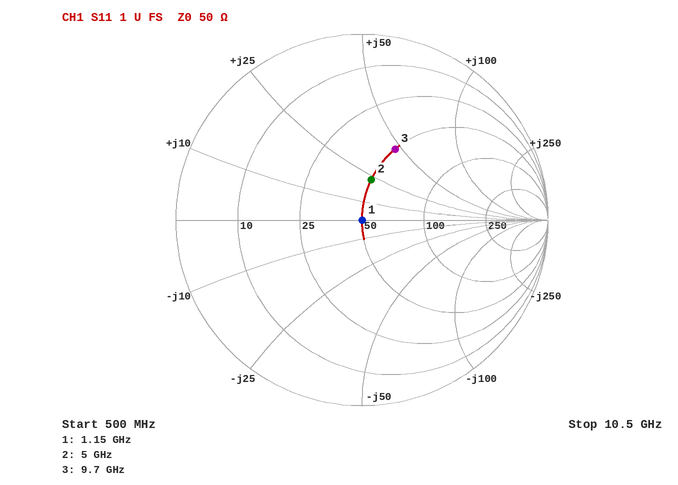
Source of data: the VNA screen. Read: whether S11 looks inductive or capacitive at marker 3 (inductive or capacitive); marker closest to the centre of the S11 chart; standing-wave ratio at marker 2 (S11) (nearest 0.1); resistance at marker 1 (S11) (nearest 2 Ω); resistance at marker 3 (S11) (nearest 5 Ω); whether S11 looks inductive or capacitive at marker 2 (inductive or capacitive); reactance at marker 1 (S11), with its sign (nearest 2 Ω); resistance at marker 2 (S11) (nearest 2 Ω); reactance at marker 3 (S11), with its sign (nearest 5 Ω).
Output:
inductive
marker 1
1.6
50 Ω
50 Ω
inductive
0 Ω
50 Ω
+45 Ω
